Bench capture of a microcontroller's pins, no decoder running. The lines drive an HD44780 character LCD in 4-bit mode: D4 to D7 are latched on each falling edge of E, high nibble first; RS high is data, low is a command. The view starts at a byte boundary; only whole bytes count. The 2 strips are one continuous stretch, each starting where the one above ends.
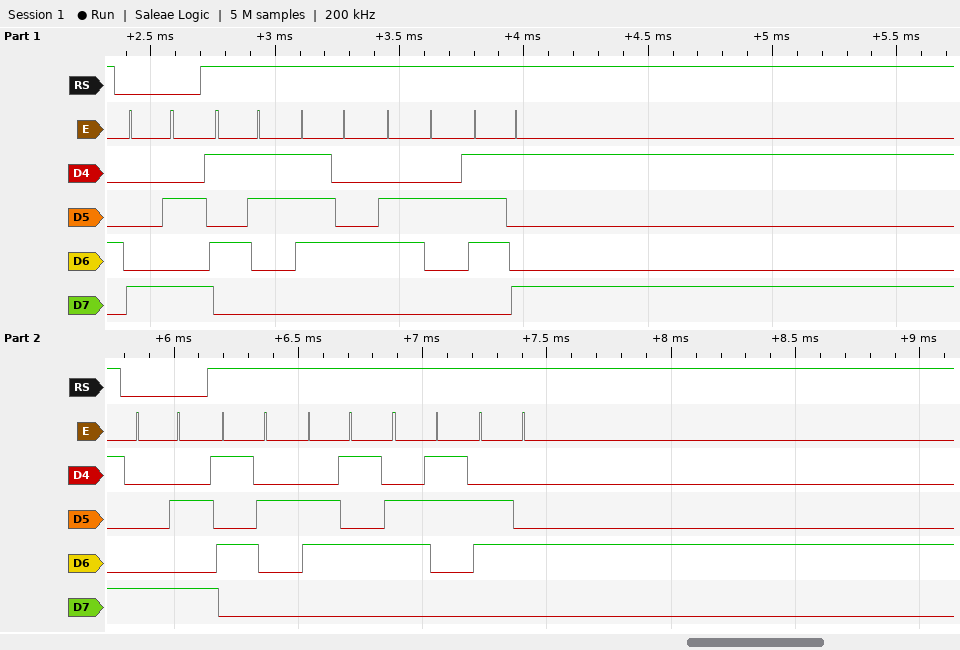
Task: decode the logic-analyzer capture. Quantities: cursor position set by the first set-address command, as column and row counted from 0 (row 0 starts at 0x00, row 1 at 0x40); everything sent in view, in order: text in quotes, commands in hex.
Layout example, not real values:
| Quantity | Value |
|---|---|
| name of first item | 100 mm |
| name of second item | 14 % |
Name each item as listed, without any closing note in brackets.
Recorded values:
| Quantity | Value |
|---|---|
| cursor position set by the first set-address command, as column and row counted from 0 | column 10, row 0 |
| everything sent in view, in order: text in quotes, commands in hex | 0x8A "Stby" 0x8A "Recd" |
